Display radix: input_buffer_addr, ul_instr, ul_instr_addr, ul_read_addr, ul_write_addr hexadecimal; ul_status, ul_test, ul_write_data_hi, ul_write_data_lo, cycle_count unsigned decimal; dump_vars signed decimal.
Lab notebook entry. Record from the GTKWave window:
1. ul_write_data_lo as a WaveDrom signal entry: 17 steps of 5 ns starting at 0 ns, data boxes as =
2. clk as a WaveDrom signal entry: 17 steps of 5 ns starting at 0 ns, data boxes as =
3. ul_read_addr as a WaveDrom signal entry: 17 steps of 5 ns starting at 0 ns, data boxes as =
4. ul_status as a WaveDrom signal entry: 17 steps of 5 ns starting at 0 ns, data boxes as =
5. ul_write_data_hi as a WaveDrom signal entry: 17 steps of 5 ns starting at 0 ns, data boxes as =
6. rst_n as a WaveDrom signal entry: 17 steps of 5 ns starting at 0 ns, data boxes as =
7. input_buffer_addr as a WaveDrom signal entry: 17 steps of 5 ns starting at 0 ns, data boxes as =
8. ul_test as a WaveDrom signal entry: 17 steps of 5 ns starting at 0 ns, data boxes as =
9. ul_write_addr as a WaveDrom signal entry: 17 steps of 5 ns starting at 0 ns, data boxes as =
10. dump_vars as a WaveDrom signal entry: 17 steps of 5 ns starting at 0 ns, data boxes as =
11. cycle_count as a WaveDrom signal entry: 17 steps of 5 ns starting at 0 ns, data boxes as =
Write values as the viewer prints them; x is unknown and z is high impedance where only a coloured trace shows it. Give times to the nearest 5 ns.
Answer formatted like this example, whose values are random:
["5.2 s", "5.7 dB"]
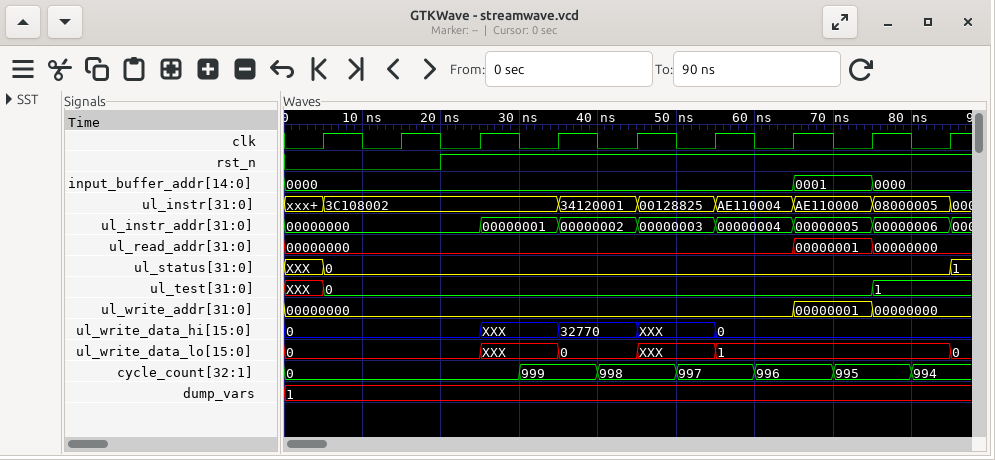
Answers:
["{name: 'ul_write_data_lo', wave: '=....x.=.x.=.....', data: '0 0 1'}", "{name: 'clk', wave: '01010101010101010'}", "{name: 'ul_read_addr', wave: '=............=.=.', data: '00000000 00000001 00000000'}", "{name: 'ul_status', wave: 'x=...............', data: '0'}", "{name: 'ul_write_data_hi', wave: '=....x.=.x.=.....', data: '0 32770 0'}", "{name: 'rst_n', wave: '0...1............'}", "{name: 'input_buffer_addr', wave: '=............=.=.', data: '0000 0001 0000'}", "{name: 'ul_test', wave: 'x=.............=.', data: '0 1'}", "{name: 'ul_write_addr', wave: '=............=.=.', data: '00000000 00000001 00000000'}", "{name: 'dump_vars', wave: '=................', data: '1'}", "{name: 'cycle_count', wave: '=.....=.=.=.=.=.=', data: '0 999 998 997 996 995 994'}"]
